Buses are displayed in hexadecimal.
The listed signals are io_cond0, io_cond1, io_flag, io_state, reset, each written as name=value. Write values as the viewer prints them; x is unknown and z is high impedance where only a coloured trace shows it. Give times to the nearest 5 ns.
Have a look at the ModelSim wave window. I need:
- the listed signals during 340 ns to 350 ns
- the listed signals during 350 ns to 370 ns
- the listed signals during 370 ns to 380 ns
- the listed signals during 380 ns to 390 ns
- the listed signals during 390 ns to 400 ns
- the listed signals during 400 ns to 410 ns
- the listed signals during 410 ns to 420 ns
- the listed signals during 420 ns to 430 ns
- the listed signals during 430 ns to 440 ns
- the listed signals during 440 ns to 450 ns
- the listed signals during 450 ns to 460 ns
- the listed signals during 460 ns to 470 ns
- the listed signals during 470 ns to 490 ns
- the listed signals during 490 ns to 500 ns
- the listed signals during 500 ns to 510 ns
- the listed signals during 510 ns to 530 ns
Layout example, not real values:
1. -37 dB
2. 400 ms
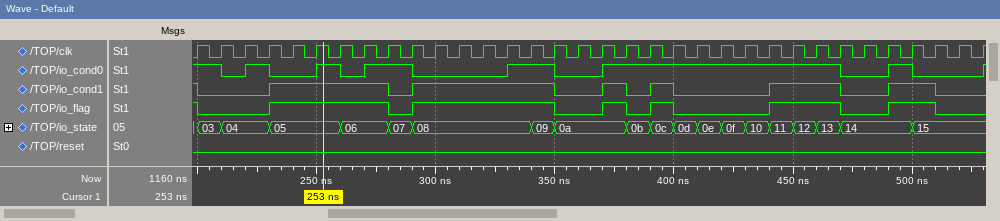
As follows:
1. io_cond0=1, io_cond1=1, io_flag=1, io_state=09, reset=0
2. io_cond0=0, io_cond1=0, io_flag=0, io_state=0a, reset=0
3. io_cond0=1, io_cond1=1, io_flag=1, io_state=0a, reset=0
4. io_cond0=1, io_cond1=0, io_flag=0, io_state=0b, reset=0
5. io_cond0=1, io_cond1=1, io_flag=1, io_state=0c, reset=0
6. io_cond0=1, io_cond1=0, io_flag=0, io_state=0d, reset=0
7. io_cond0=1, io_cond1=0, io_flag=0, io_state=0e, reset=0
8. io_cond0=1, io_cond1=0, io_flag=0, io_state=0f, reset=0
9. io_cond0=1, io_cond1=0, io_flag=0, io_state=10, reset=0
10. io_cond0=1, io_cond1=1, io_flag=1, io_state=11, reset=0
11. io_cond0=1, io_cond1=1, io_flag=1, io_state=12, reset=0
12. io_cond0=1, io_cond1=1, io_flag=1, io_state=13, reset=0
13. io_cond0=0, io_cond1=0, io_flag=0, io_state=14, reset=0
14. io_cond0=1, io_cond1=1, io_flag=1, io_state=14, reset=0
15. io_cond0=0, io_cond1=1, io_flag=1, io_state=15, reset=0
16. io_cond0=0, io_cond1=0, io_flag=0, io_state=15, reset=0
